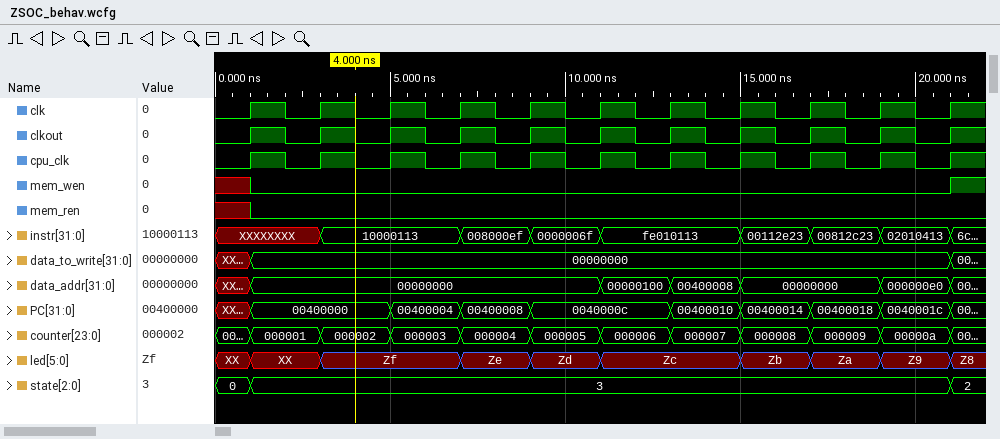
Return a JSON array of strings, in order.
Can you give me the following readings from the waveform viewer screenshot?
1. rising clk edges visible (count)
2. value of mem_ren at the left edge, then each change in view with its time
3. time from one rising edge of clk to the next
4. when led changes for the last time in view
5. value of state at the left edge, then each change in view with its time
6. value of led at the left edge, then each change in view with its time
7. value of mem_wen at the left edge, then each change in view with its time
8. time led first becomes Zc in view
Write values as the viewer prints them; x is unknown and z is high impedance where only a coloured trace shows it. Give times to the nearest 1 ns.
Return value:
["11", "x, 0 at 1 ns", "2 ns", "21 ns", "0, 3 at 1 ns, 2 at 21 ns", "XX, XX at 1 ns, Zf at 3 ns, Ze at 7 ns, Zd at 9 ns, Zc at 11 ns, Zb at 15 ns, Za at 17 ns, Z9 at 19 ns, Z8 at 21 ns", "x, 0 at 1 ns, 1 at 21 ns", "11 ns"]
